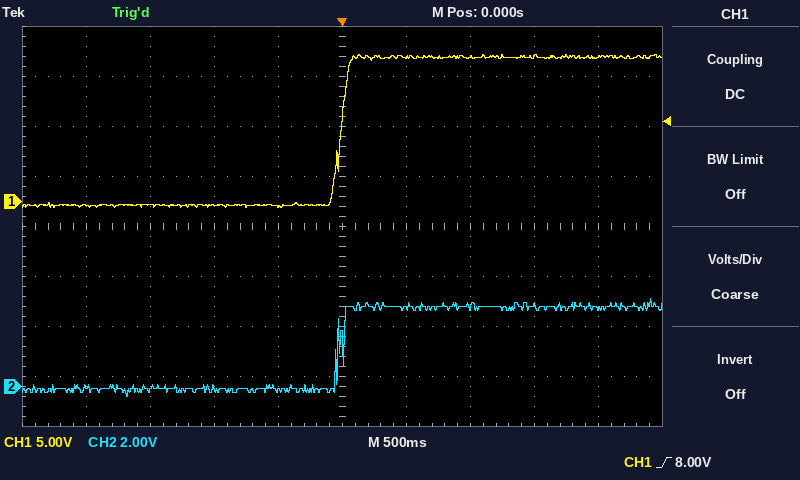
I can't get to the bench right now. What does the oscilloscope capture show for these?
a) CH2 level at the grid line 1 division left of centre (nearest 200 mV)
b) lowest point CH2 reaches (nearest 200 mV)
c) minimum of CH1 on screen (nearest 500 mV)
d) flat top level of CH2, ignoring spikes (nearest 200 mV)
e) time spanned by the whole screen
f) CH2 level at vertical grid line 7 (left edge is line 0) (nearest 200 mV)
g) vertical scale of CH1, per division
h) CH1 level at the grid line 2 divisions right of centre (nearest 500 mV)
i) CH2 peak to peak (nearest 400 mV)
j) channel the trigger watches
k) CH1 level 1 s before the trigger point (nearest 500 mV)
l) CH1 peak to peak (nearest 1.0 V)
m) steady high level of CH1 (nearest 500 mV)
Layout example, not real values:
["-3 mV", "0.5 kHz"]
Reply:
["-200 mV", "-400 mV", "-500 mV", "3.2 V", "5 s", "3.2 V", "5 V", "14.5 V", "4.0 V", "CH1", "-500 mV", "15.0 V", "14.5 V"]
